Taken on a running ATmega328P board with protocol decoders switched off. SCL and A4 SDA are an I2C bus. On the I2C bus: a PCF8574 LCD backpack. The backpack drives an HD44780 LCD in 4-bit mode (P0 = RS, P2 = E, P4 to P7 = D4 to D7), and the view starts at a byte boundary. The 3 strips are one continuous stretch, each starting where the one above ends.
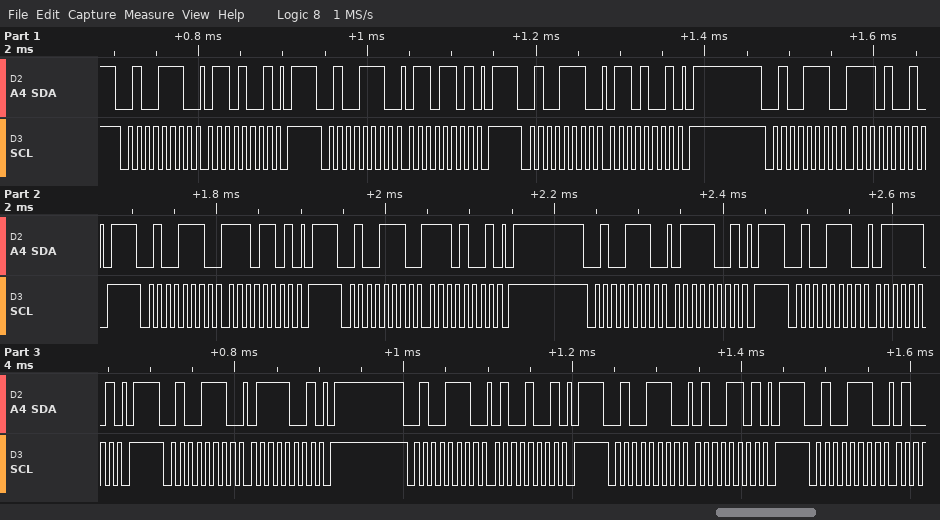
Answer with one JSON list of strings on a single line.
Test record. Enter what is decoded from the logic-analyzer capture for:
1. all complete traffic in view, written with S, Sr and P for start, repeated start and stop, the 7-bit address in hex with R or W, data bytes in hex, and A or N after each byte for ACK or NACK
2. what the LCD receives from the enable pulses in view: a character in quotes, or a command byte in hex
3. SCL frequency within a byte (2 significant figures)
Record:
["S 27W A 69 A P S 27W A 6D A P S 27W A 69 A P S 27W A E9 A P S 27W A ED A P S 27W A E9 A P S 27W A 79 A P S 27W A 7D A P S 27W A 79 A P S 27W A 49 A P S 27W A 4D A P S 27W A", "'n'", "100 kHz"]
